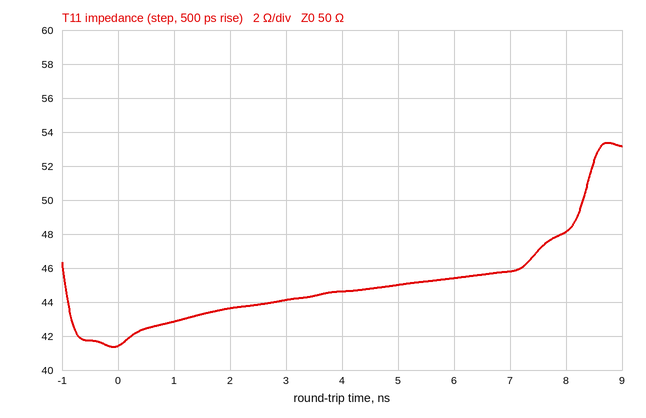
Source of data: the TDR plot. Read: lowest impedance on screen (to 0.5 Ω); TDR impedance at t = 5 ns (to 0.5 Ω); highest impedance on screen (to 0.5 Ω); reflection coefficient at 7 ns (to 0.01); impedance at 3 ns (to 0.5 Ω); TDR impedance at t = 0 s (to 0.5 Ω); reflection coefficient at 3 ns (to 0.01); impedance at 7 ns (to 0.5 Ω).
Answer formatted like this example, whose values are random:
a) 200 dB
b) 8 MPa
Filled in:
a) 41.5 Ω
b) 45.0 Ω
c) 53.5 Ω
d) -0.04
e) 44.0 Ω
f) 41.5 Ω
g) -0.06
h) 46.0 Ω
